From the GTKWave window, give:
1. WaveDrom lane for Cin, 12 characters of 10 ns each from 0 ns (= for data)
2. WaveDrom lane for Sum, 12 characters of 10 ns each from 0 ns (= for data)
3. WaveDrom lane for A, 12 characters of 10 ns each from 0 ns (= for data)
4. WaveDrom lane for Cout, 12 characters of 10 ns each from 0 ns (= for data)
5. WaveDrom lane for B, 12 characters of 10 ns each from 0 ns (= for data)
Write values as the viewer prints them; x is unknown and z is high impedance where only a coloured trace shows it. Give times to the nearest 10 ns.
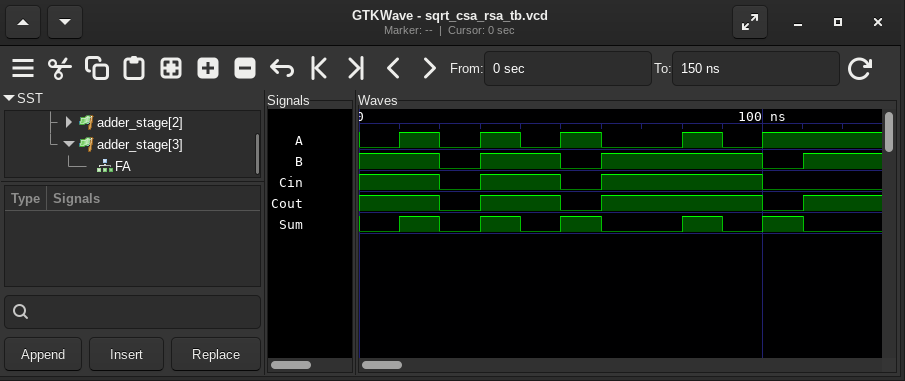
{name: 'Cin', wave: '1.01.01...0.'}
{name: 'Sum', wave: '0101010.1010'}
{name: 'A', wave: '0101010.101.'}
{name: 'Cout', wave: '1.01.01...01'}
{name: 'B', wave: '1.01.01...01'}
